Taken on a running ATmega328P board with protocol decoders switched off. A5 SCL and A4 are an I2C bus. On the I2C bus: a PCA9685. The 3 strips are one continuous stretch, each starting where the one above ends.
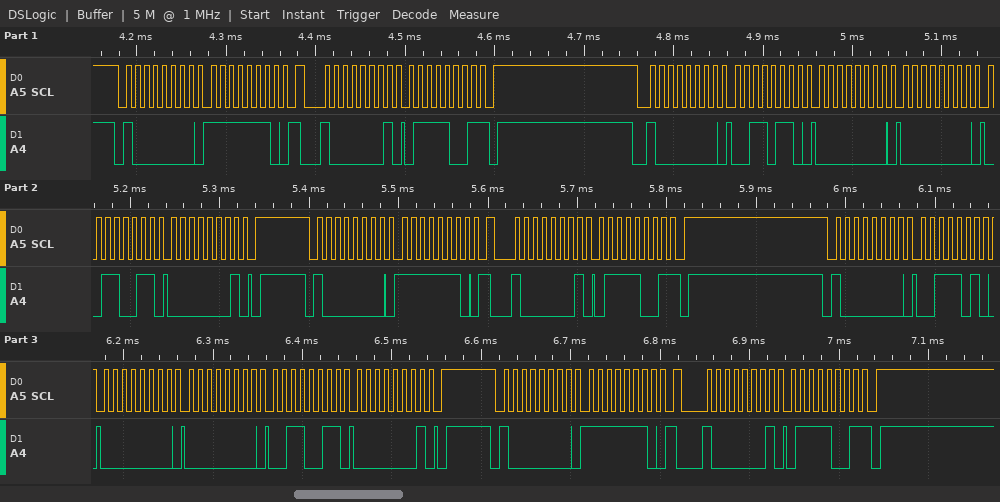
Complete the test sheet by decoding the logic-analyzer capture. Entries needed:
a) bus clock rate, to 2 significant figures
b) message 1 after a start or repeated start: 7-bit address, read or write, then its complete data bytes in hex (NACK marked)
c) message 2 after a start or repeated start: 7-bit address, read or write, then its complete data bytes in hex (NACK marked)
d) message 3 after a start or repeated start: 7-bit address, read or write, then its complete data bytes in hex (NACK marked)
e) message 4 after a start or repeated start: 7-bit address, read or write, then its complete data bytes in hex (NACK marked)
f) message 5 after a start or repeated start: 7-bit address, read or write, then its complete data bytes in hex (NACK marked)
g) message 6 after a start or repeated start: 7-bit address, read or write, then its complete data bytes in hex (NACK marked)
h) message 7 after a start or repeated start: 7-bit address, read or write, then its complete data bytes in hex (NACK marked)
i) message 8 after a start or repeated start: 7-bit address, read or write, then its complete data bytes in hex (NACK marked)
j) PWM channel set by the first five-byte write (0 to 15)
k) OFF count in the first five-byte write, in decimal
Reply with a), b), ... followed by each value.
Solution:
a) 100 kHz
b) 0x40 write: FE
c) 0x40 read: 79 NACK
d) 0x40 write: 36 00 00 33 01
e) 0x40 write: FE
f) 0x40 read: 79 NACK
g) 0x40 write: 3A 00 00 33 01
h) 0x40 write: FE
i) 0x40 read: 79 NACK
j) 12
k) 307
